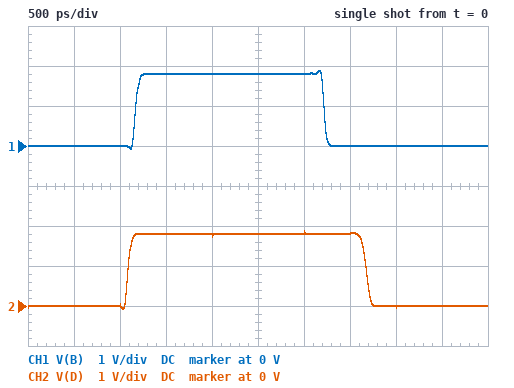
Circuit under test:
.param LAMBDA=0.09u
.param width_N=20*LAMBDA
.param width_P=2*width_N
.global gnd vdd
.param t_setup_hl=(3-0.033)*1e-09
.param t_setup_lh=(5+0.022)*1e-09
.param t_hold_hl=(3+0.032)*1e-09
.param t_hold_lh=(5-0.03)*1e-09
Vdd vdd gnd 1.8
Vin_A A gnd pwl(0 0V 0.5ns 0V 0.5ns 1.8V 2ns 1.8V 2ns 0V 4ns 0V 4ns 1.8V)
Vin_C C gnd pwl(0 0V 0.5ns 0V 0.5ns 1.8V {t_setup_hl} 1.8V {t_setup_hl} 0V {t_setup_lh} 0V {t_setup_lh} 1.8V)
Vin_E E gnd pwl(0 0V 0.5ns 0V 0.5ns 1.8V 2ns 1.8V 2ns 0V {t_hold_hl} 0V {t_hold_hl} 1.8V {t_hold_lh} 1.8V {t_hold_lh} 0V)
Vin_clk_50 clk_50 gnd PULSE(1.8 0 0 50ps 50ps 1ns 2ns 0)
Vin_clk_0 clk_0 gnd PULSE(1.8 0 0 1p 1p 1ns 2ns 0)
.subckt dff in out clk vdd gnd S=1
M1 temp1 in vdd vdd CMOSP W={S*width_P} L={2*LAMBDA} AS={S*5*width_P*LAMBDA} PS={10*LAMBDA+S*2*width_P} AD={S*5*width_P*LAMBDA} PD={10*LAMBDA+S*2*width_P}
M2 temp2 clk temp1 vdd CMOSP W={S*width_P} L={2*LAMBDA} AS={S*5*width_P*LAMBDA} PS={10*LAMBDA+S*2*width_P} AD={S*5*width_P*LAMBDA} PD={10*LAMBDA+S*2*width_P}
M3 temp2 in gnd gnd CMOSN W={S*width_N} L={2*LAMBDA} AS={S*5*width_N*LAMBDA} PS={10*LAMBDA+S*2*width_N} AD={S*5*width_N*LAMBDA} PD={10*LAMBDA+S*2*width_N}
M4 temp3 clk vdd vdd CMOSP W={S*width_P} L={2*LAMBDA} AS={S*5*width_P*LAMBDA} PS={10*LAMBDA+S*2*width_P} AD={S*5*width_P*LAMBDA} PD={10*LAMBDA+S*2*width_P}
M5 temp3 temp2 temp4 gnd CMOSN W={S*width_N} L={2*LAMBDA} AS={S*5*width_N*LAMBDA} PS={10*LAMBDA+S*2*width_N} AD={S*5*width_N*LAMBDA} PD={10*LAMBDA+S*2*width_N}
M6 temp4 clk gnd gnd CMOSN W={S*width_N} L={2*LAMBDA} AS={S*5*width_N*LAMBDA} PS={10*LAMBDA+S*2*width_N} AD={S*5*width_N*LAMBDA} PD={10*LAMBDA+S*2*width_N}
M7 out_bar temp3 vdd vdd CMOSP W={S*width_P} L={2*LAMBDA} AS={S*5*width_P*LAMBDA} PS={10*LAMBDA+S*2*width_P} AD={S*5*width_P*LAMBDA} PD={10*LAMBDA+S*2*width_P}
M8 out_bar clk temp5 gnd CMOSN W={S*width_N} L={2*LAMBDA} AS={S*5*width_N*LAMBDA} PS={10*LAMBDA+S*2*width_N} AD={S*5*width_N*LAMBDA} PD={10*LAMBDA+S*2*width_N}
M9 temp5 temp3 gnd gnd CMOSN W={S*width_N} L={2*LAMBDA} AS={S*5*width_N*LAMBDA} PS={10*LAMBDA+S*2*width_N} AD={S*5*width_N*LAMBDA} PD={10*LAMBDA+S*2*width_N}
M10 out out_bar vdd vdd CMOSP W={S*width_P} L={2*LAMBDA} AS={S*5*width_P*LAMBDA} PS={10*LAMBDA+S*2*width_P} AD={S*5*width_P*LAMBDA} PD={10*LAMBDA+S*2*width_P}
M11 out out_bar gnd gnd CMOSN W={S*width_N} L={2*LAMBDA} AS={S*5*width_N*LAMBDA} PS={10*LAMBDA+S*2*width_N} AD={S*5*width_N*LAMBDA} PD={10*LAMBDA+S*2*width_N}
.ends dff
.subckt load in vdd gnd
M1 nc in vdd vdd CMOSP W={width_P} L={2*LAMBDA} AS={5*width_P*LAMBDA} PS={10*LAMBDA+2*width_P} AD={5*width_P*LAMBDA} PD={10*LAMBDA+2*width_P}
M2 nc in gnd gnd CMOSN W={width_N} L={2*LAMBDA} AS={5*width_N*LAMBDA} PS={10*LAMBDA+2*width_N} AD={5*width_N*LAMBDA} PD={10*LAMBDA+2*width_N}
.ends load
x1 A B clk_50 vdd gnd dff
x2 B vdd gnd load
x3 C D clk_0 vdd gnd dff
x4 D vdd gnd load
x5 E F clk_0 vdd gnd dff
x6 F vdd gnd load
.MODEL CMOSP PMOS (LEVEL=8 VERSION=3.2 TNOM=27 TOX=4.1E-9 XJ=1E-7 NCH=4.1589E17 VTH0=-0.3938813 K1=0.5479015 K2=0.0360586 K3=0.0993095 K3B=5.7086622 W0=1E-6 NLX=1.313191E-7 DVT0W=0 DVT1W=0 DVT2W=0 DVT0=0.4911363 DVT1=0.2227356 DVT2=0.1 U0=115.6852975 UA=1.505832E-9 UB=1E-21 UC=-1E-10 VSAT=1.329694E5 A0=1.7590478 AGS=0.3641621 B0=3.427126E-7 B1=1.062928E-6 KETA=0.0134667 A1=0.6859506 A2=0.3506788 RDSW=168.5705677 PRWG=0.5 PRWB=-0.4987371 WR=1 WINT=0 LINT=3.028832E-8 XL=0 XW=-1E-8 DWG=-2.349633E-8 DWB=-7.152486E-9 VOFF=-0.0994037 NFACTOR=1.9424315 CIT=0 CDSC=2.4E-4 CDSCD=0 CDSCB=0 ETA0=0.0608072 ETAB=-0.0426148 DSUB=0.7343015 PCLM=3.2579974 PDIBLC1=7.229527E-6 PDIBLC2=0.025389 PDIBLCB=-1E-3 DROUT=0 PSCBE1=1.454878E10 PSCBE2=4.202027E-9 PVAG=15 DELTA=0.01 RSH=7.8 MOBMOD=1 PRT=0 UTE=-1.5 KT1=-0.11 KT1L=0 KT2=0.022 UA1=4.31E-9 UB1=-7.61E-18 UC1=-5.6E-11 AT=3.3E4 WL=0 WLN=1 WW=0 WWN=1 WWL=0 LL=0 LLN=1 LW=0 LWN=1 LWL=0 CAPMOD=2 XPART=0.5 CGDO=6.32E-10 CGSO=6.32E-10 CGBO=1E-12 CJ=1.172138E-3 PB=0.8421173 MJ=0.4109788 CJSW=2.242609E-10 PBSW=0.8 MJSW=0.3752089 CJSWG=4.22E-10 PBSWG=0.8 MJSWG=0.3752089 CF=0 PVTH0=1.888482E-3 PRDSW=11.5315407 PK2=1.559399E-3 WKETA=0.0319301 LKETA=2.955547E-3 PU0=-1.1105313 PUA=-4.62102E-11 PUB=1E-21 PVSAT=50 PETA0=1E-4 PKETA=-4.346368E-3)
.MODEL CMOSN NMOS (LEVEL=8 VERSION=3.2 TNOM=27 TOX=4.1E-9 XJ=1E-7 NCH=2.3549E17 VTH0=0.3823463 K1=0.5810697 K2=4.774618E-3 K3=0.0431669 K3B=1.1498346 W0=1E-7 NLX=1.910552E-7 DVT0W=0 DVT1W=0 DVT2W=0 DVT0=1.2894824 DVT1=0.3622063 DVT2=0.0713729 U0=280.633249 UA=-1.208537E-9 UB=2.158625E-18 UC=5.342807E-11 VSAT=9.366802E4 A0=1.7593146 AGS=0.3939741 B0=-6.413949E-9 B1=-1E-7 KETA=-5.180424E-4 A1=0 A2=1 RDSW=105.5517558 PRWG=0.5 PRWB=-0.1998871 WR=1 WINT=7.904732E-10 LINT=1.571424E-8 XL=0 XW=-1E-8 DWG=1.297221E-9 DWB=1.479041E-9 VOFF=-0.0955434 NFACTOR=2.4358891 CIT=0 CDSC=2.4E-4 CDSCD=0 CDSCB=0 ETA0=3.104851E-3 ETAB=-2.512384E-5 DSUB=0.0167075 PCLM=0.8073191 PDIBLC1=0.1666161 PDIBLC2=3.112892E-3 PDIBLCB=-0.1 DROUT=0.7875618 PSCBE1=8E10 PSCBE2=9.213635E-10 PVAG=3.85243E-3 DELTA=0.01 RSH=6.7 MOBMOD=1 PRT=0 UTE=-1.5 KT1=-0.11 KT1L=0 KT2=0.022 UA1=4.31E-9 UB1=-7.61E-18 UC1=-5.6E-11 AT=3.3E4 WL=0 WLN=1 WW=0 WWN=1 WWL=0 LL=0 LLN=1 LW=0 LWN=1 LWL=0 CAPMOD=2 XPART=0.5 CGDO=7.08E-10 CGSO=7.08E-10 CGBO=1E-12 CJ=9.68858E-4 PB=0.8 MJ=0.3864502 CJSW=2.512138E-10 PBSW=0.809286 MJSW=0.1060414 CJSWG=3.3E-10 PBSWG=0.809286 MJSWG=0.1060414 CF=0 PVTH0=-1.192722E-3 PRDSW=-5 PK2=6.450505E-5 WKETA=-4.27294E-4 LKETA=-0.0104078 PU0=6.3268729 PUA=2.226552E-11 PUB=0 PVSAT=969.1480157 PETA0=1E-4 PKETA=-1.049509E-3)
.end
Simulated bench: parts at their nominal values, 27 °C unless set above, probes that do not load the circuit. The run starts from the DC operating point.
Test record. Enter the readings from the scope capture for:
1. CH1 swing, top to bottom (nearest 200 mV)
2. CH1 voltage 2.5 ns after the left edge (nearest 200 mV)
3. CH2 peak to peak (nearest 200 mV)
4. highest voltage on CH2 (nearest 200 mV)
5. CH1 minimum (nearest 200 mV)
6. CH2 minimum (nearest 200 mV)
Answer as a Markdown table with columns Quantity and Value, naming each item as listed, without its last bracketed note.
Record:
| Quantity | Value |
|---|---|
| CH1 swing, top to bottom | 2.0 V |
| CH1 voltage 2.5 ns after the left edge | 1.8 V |
| CH2 peak to peak | 2.0 V |
| highest voltage on CH2 | 1.8 V |
| CH1 minimum | 0 V |
| CH2 minimum | 0 V |
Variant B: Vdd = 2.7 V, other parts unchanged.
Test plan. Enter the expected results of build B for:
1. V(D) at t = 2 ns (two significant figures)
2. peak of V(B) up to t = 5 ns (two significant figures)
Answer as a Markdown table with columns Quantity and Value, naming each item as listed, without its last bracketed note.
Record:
| Quantity | Value |
|---|---|
| V(D) at t = 2 ns | 2.7 V |
| peak of V(B) up to t = 5 ns | 2.8 V |
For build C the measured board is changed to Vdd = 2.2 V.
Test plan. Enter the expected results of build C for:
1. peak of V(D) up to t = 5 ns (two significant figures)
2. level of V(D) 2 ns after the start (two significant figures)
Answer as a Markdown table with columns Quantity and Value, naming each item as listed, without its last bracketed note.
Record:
| Quantity | Value |
|---|---|
| peak of V(D) up to t = 5 ns | 2.3 V |
| level of V(D) 2 ns after the start | 2.2 V |
